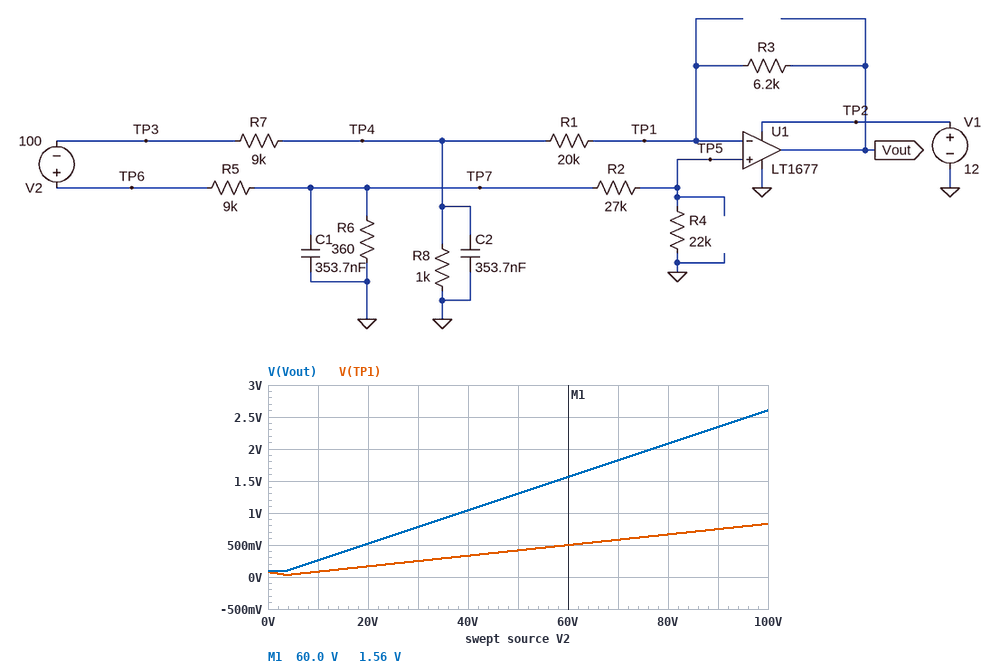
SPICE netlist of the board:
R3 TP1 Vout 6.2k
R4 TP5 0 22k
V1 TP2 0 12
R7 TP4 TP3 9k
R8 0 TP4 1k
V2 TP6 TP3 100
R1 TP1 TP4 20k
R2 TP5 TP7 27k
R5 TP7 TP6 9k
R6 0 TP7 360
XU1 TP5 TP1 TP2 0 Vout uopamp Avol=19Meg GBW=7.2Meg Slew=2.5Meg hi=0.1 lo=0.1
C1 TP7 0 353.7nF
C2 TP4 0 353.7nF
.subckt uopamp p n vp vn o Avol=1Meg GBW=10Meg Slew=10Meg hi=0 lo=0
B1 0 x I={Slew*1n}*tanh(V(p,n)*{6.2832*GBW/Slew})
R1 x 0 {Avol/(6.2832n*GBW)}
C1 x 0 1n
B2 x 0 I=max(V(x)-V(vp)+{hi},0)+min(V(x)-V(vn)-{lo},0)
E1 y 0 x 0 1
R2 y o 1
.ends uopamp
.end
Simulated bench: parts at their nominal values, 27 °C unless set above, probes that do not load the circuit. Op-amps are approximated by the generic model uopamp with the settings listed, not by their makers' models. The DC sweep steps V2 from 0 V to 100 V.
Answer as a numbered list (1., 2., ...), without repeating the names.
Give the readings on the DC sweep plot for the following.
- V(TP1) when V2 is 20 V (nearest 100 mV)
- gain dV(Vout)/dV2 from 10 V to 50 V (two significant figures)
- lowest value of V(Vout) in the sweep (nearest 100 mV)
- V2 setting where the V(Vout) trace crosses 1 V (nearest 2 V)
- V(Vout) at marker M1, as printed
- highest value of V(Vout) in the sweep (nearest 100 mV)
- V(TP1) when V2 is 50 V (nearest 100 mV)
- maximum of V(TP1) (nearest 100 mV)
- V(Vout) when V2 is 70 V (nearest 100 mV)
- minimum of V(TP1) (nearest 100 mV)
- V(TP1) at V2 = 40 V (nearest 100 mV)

1. 200 mV
2. 0.026 V/V
3. 100 mV
4. 38 V
5. 1.56 V
6. 2.6 V
7. 400 mV
8. 800 mV
9. 1.8 V
10. 0 V
11. 300 mV
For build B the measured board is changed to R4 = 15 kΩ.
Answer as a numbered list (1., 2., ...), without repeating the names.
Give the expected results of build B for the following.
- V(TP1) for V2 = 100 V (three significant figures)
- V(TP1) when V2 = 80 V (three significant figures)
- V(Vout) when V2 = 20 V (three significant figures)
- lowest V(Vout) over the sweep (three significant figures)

1. 660 mV
2. 528 mV
3. 477 mV
4. 97.8 mV
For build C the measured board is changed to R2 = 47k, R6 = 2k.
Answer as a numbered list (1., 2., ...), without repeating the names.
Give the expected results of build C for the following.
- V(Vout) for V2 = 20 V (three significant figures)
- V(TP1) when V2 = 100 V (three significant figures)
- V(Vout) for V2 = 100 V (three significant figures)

1. 1.05 V
2. 2.97 V
3. 5.26 V
